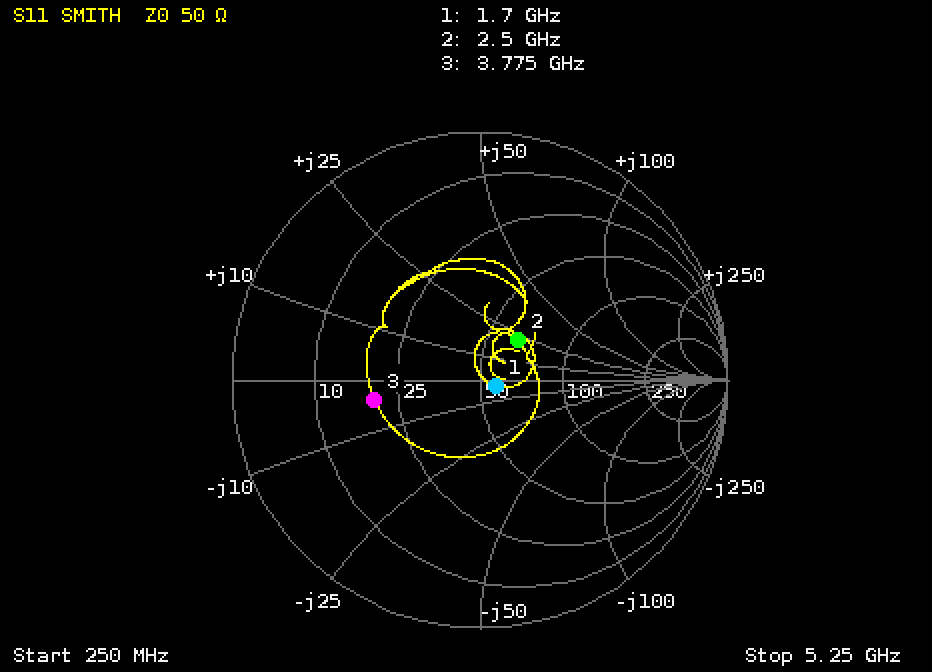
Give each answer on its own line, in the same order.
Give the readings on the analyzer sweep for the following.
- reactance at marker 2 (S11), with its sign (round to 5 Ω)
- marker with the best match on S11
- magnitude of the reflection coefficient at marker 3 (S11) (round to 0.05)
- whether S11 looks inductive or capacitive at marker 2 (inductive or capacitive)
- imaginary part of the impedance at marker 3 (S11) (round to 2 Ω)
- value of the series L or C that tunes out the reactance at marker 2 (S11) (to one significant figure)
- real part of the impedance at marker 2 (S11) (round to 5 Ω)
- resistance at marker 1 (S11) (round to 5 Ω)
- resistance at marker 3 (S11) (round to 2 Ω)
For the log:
+20 Ω
marker 1
0.45
inductive
-4 Ω
3 pF
65 Ω
55 Ω
20 Ω
